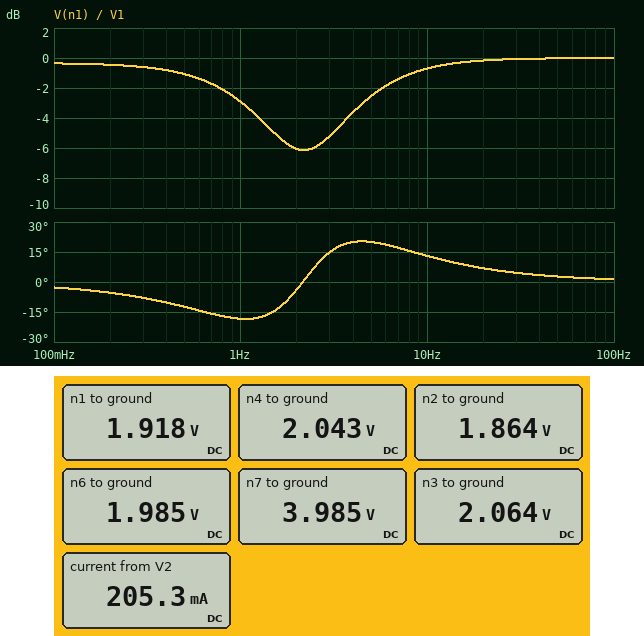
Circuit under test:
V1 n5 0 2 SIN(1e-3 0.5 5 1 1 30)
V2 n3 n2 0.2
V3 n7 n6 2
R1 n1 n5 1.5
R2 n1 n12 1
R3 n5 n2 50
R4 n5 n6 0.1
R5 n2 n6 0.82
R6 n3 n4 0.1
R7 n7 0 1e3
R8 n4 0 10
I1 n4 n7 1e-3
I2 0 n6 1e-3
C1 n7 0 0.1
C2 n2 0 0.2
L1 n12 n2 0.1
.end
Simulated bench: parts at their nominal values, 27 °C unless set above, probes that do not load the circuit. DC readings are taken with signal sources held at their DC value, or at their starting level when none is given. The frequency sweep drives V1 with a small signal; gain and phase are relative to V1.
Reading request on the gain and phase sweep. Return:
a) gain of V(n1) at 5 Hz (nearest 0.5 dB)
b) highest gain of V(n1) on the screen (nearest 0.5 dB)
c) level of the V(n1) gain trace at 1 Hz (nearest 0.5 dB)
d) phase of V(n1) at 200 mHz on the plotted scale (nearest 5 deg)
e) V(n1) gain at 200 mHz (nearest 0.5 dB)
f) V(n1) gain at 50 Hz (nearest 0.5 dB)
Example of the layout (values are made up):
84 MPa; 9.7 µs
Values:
-2.5 dB; 0 dB; -3.0 dB; -5 deg; -0.5 dB; 0 dB
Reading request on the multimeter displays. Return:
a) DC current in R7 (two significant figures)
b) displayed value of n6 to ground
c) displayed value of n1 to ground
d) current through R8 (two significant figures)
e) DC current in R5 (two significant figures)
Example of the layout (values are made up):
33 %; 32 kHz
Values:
4.0 mA; 1.985 V; 1.918 V; 200 mA; 150 mA
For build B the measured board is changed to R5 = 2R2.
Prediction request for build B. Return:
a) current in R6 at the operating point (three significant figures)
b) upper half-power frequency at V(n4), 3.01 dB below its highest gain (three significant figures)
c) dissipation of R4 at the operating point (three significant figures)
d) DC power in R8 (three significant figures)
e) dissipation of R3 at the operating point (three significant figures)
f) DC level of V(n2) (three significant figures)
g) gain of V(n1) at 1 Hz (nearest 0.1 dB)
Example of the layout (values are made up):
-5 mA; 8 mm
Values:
196 mA; 814 mHz; 1.03 mW; 381 mW; 1.05 mW; 1.77 V; -5.1 dB
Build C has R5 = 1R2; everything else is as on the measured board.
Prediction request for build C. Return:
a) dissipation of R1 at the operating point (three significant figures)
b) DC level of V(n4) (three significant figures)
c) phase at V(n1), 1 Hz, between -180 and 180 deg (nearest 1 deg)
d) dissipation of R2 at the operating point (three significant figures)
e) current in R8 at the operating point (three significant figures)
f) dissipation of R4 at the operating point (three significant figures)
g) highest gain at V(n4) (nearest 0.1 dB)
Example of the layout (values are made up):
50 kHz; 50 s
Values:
6.93 mW; 2.01 V; -19 deg; 4.62 mW; 201 mA; 1.76 mW; -0.8 dB
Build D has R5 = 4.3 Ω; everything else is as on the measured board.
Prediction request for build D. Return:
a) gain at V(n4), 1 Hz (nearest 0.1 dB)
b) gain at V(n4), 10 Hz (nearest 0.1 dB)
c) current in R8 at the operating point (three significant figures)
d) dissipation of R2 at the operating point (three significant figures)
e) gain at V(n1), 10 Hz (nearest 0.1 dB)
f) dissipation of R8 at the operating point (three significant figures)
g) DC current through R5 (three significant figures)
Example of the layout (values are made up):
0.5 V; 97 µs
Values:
-6.8 dB; -31.4 dB; 189 mA; 13.8 mW; -0.6 dB; 356 mW; 66.6 mA
